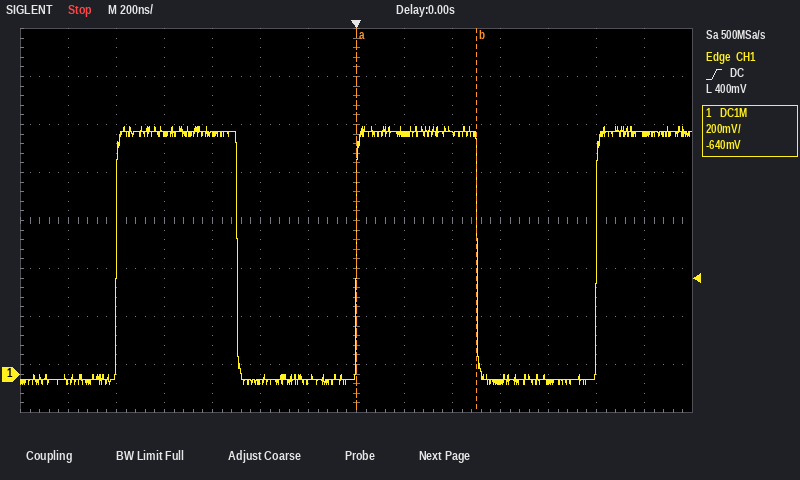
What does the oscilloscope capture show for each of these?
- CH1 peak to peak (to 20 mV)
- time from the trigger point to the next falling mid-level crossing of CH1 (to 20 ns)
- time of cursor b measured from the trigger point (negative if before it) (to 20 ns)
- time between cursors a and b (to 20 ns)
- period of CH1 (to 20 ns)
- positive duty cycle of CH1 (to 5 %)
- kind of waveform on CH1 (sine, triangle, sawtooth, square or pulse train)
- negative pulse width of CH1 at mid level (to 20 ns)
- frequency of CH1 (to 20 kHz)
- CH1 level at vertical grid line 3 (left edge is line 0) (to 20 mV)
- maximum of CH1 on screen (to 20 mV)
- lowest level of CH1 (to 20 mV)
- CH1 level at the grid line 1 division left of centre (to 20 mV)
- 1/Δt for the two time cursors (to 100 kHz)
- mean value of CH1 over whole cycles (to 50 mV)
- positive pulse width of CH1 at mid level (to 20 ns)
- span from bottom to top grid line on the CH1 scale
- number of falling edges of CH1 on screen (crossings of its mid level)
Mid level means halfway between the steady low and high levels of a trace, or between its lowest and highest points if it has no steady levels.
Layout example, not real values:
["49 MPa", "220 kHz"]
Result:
["1.08 V", "500 ns", "+500 ns", "500 ns", "1.00 µs", "50 %", "square", "500 ns", "1.00 MHz", "1.00 V", "1.04 V", "-40 mV", "-40 mV", "2.0 MHz", "500 mV", "500 ns", "1.6 V", "2"]
